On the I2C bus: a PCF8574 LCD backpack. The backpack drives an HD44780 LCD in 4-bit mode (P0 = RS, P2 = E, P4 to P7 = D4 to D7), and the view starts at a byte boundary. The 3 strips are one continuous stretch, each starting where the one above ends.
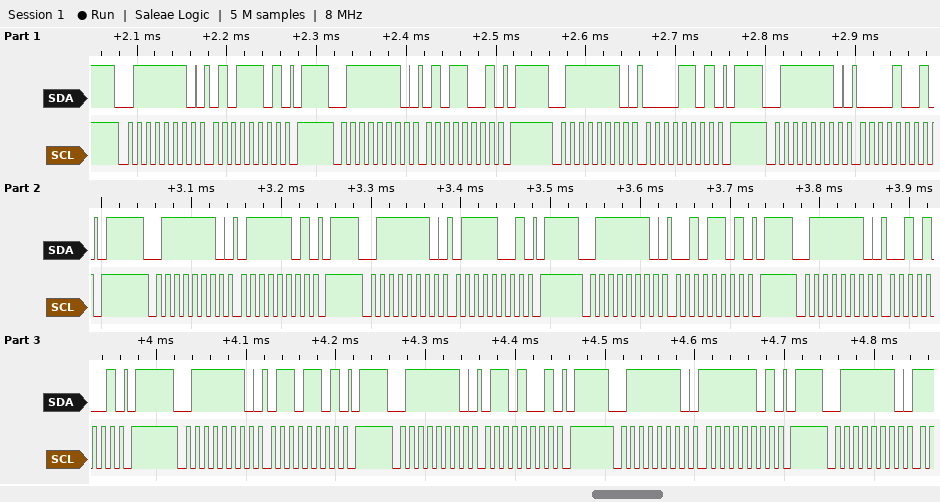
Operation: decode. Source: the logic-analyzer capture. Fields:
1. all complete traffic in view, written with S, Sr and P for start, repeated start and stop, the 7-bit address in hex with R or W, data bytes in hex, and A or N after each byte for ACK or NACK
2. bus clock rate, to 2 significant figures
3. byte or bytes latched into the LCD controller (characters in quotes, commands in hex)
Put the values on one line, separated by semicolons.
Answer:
S 3FW A 5D A P S 3FW A 59 A P S 3FW A 0D A P S 3FW A 09 A P S 3FW A 7D A P S 3FW A 79 A P S 3FW A 2D A P S 3FW A 29 A P S 3FW A 6D A P S 3FW A 69 A P S 3FW A FD A P S 3FW A; 100 kHz; 'P' 'r'
